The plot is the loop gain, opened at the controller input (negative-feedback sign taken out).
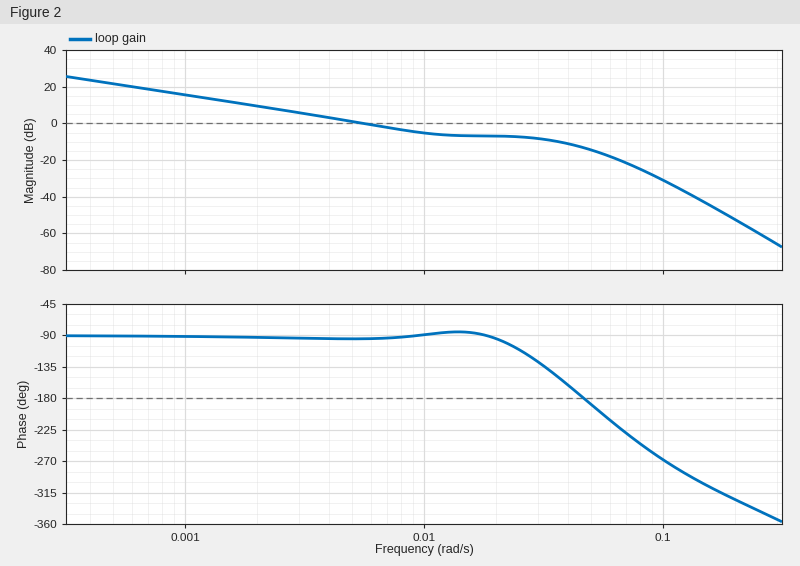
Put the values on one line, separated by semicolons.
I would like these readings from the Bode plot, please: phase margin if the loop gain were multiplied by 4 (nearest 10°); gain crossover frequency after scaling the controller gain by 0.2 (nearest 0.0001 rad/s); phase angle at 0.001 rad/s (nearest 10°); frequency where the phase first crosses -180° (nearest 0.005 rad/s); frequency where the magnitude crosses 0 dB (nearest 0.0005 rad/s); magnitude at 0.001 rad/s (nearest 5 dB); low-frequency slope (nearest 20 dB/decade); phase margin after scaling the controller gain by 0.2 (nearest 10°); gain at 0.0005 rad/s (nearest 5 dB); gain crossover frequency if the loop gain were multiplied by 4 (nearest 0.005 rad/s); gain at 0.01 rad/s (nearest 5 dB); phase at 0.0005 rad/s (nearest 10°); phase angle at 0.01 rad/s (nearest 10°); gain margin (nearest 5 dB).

10°; 0.0012 rad/s; -90°; 0.045 rad/s; 0.0055 rad/s; 15 dB; -20 dB/decade; 90°; 20 dB; 0.045 rad/s; -5 dB; -90°; -90°; 15 dB
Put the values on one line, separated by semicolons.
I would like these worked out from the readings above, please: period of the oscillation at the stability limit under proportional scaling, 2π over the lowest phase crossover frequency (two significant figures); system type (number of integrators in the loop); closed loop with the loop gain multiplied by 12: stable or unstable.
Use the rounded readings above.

140 s; 1; unstable
